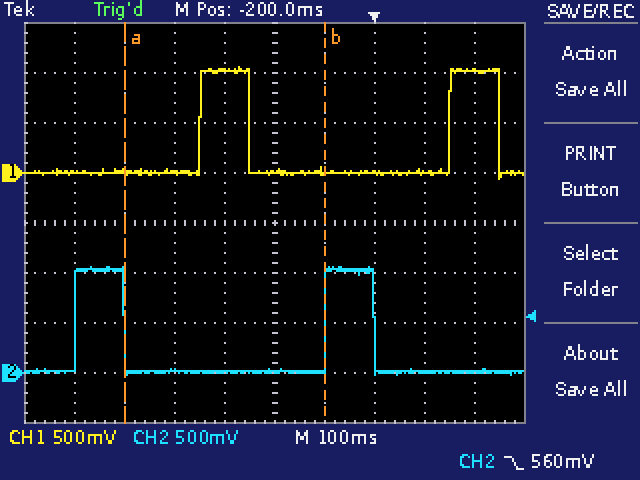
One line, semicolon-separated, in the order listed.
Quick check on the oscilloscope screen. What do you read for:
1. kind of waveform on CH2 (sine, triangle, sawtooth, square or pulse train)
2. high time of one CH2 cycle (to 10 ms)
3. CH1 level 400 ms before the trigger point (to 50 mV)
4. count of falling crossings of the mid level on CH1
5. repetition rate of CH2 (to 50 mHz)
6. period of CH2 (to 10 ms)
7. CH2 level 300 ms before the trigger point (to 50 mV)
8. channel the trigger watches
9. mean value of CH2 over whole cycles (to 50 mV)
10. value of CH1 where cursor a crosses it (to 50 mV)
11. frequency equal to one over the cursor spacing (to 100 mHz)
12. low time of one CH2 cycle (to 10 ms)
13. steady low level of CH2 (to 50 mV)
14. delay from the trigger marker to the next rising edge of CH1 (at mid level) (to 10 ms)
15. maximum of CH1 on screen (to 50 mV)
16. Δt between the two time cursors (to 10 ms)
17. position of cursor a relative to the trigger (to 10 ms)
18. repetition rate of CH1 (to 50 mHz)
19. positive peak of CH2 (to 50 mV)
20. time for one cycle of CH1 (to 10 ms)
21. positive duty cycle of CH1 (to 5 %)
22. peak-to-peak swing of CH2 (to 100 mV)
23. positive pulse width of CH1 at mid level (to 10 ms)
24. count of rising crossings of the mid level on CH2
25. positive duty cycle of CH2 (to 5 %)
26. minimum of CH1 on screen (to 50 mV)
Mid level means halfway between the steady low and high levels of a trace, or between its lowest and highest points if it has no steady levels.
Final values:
pulse train; 100 ms; 0 mV; 2; 2.00 Hz; 500 ms; 0 mV; CH2; 200 mV; 0 mV; 2.5 Hz; 400 ms; 0 mV; 150 ms; 1.05 V; 400 ms; -500 ms; 2.00 Hz; 1.05 V; 500 ms; 20 %; 1.10 V; 100 ms; 2; 20 %; -50 mV
